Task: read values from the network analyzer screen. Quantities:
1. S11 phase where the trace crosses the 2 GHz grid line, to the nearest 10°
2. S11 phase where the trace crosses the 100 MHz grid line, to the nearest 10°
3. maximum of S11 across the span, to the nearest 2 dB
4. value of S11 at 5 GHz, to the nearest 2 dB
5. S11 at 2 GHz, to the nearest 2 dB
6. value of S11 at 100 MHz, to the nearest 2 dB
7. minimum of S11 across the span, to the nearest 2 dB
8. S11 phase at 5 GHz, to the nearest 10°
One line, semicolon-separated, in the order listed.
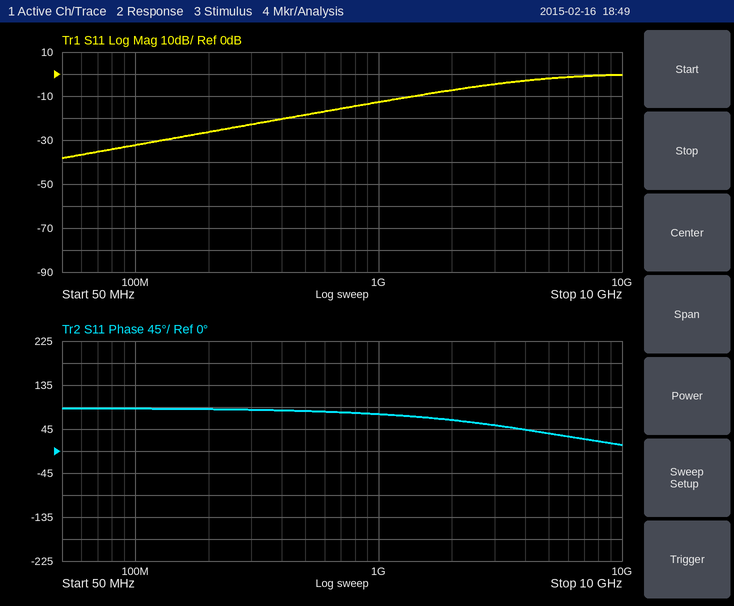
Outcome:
60°; 90°; 0 dB; -2 dB; -8 dB; -32 dB; -38 dB; 40°
